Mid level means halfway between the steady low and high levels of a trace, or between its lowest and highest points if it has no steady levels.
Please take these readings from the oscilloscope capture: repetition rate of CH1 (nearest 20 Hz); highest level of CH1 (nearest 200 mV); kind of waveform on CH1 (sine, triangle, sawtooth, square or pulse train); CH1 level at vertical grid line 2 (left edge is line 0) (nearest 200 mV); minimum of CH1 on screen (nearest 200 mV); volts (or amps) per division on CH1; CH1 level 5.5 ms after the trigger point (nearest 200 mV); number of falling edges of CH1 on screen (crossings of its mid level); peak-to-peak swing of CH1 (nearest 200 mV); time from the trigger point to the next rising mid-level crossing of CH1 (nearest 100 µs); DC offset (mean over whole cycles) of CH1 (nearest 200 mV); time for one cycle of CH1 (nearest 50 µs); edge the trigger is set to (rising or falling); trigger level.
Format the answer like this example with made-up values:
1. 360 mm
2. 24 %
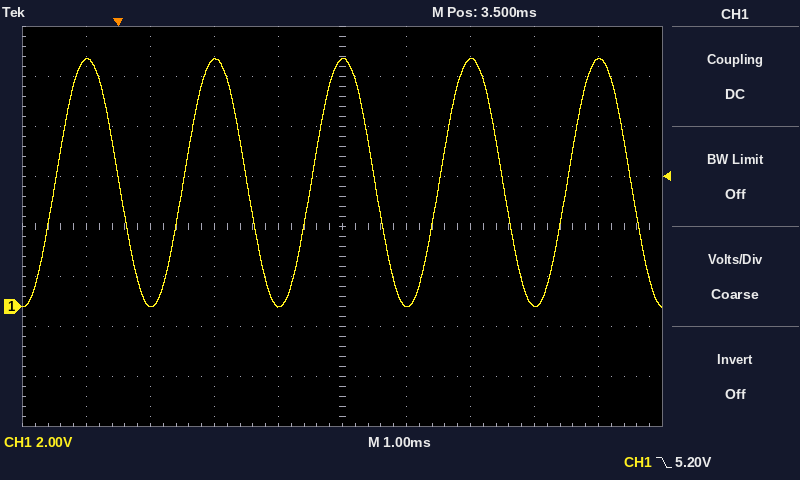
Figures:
1. 500 Hz
2. 10.0 V
3. sine
4. 0.0 V
5. 0.0 V
6. 2 V
7. 9.8 V
8. 5
9. 10.0 V
10. 1.0 ms
11. 5.0 V
12. 2.00 ms
13. falling
14. 5.20 V
